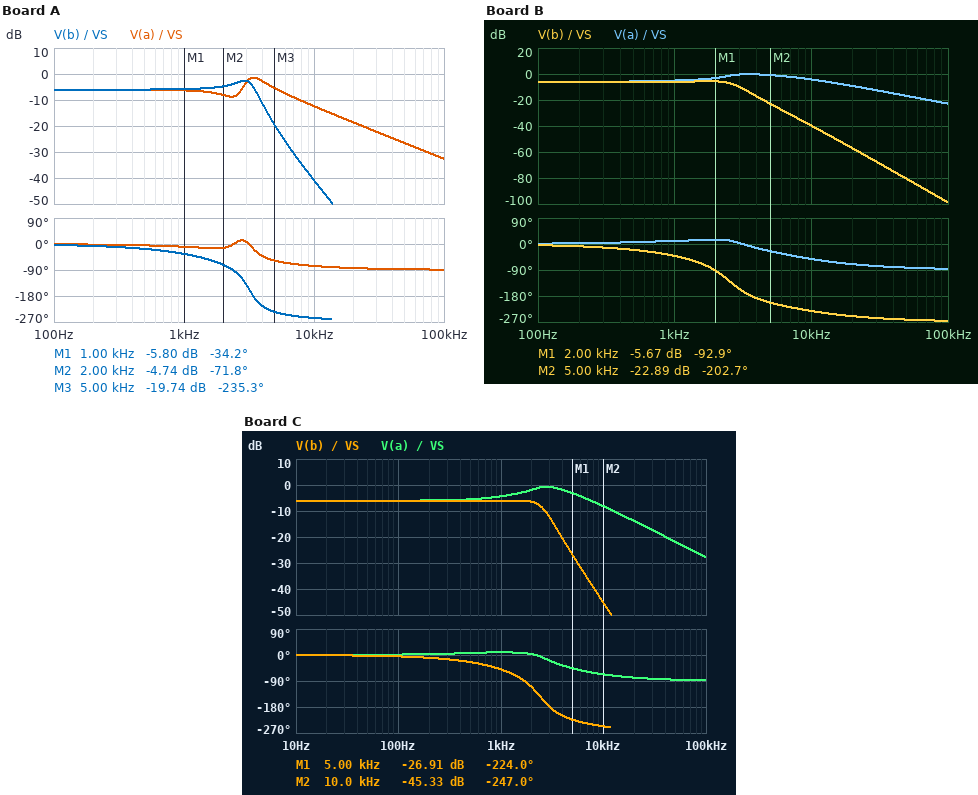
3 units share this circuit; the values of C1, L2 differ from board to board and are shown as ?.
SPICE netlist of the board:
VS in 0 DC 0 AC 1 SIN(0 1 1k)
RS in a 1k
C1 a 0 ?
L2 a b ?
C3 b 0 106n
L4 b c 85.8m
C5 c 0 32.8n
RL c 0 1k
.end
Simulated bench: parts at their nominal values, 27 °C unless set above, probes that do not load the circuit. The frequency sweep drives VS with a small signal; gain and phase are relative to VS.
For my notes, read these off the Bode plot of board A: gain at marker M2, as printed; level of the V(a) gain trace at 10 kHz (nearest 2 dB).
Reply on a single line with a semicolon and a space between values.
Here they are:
-4.74 dB; -12 dB
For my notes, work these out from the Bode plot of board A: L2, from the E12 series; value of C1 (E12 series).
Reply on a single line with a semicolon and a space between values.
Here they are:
68 mH; 68 nF
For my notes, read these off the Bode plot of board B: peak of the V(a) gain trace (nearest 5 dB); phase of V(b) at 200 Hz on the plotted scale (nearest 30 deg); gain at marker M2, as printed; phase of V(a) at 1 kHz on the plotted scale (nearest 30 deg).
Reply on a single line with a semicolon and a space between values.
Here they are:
0 dB; 0 deg; -22.89 dB; 0 deg
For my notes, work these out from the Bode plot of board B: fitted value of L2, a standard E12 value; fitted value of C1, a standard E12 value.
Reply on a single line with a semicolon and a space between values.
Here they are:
150 mH; 22 nF
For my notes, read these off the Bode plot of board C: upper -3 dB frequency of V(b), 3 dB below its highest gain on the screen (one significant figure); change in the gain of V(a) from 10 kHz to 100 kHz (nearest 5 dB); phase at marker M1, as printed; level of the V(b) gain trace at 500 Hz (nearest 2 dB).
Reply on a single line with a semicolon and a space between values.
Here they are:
3 kHz; -20 dB; -224.0 deg; -6 dB
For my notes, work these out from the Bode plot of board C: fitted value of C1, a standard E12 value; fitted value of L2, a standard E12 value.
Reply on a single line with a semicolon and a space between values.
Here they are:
39 nF; 180 mH
